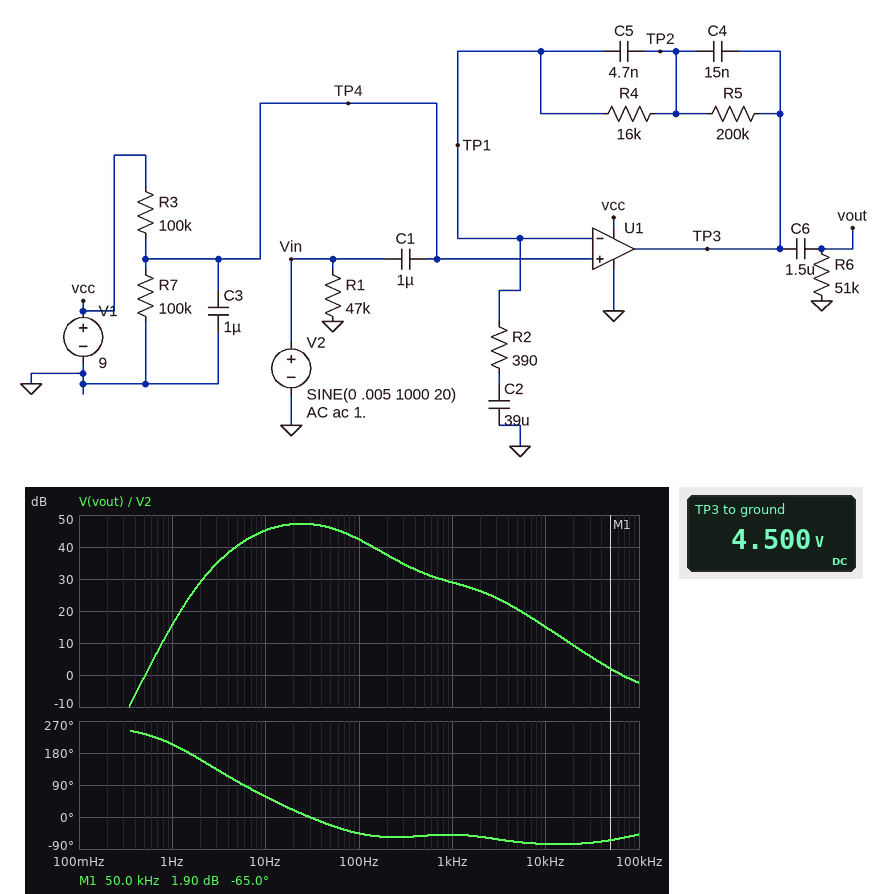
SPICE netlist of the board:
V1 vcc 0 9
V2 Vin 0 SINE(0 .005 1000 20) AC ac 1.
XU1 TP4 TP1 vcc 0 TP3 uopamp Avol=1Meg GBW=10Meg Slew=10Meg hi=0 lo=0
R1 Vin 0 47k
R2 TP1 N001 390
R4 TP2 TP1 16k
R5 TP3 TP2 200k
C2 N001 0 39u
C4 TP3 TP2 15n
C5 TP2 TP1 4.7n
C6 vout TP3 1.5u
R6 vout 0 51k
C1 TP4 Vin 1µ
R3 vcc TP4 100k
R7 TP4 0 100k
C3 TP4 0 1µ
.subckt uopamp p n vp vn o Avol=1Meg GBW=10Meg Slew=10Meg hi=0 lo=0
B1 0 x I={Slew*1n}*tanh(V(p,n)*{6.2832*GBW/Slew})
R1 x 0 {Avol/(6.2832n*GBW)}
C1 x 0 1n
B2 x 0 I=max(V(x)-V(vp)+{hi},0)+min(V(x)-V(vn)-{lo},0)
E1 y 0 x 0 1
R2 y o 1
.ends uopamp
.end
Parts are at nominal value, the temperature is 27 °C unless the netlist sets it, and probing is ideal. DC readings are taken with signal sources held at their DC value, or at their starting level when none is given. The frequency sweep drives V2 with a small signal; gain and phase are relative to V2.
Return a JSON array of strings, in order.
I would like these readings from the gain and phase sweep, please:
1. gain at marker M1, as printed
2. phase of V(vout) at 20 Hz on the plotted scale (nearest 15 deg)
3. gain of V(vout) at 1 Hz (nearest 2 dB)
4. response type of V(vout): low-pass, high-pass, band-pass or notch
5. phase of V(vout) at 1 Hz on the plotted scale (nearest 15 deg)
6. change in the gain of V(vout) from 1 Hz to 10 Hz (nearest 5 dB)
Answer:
["1.90 dB", "15 deg", "16 dB", "band-pass", "210 deg", "30 dB"]
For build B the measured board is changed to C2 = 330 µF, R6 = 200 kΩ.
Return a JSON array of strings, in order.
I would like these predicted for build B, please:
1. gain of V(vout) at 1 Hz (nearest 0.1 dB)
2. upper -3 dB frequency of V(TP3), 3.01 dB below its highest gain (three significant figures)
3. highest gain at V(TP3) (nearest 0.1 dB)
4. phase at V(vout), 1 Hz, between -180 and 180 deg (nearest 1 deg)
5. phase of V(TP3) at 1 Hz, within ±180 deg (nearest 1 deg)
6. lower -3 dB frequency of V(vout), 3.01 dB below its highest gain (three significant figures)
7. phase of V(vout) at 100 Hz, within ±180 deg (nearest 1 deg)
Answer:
["38.3 dB", "57.4 Hz", "48.5 dB", "136 deg", "108 deg", "2.17 Hz", "-52 deg"]
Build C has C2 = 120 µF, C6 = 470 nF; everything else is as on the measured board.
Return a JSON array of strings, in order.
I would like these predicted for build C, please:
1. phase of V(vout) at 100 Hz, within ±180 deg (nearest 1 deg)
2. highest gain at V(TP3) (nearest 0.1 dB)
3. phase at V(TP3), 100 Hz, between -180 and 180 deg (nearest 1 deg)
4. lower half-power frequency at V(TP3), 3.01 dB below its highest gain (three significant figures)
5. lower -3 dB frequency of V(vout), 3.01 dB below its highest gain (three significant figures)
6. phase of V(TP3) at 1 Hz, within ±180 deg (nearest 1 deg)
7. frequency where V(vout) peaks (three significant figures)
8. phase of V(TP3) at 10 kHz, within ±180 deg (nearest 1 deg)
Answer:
["-48 deg", "48.3 dB", "-51 deg", "3.57 Hz", "6.79 Hz", "130 deg", "20.4 Hz", "-76 deg"]
